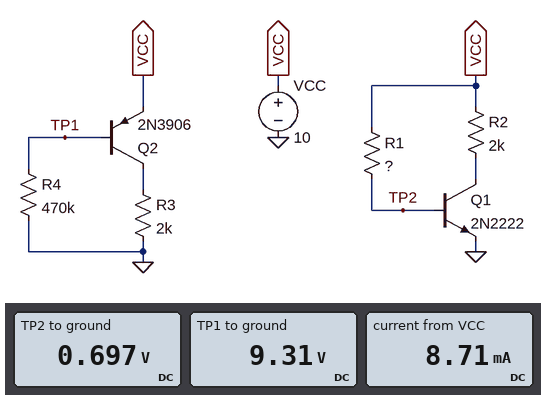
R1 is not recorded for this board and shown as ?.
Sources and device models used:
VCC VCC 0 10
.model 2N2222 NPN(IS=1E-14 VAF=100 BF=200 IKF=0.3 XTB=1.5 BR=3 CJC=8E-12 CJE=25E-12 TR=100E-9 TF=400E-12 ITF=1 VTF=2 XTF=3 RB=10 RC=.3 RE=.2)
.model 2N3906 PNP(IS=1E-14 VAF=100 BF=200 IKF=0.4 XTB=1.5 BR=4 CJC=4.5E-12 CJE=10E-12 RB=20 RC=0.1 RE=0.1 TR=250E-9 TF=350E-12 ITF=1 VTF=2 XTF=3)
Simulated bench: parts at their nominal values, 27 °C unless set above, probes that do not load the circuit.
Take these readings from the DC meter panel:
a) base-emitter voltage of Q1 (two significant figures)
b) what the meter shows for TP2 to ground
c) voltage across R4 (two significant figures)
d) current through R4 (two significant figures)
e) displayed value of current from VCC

700 mV
0.697 V
9.3 V
20 µA
8.71 mA
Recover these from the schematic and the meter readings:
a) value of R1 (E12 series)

390 kΩ
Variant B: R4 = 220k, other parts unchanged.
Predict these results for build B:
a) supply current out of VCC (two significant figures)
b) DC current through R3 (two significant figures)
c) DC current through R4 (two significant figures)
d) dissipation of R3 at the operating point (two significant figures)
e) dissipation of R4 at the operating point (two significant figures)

9.7 mA
4.9 mA
42 µA
49 mW
390 µW
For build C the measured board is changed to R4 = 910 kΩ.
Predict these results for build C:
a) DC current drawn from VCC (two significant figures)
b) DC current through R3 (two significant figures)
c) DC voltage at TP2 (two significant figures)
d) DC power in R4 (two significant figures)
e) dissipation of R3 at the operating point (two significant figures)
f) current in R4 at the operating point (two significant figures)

6.9 mA
2.1 mA
700 mV
96 µW
9.2 mW
10 µA
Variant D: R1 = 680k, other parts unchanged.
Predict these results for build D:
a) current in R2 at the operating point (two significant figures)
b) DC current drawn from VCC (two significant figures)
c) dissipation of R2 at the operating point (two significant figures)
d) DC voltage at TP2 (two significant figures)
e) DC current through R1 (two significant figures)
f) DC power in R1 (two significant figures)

2.8 mA
6.8 mA
16 mW
680 mV
14 µA
130 µW
